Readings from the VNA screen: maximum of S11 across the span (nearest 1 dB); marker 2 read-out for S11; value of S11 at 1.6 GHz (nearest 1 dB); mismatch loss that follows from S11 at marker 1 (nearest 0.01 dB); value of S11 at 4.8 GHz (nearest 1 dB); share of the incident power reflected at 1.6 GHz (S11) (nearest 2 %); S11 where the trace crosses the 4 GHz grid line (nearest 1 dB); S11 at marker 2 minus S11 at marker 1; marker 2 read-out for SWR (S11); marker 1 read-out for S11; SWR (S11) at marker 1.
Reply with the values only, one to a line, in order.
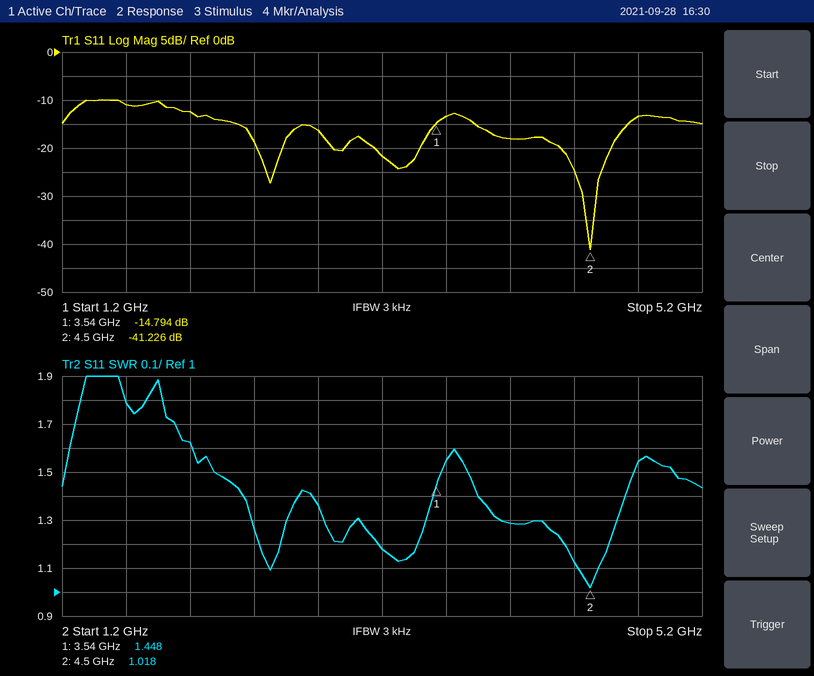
-10 dB
-41.226 dB
-11 dB
0.15 dB
-13 dB
8 %
-18 dB
-26.432 dB
1.018
-14.794 dB
1.448
